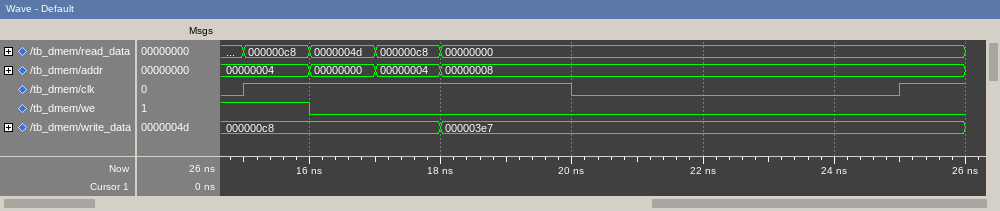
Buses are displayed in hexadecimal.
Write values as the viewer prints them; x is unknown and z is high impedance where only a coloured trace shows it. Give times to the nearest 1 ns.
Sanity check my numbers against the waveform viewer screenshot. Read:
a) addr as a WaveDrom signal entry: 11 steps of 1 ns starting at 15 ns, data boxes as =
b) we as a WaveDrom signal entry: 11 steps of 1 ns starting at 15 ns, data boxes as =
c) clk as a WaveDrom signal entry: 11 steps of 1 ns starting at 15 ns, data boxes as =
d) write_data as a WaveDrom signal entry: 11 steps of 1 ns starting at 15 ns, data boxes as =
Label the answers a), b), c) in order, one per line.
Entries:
a) {name: 'addr', wave: '====.......', data: '00000004 00000000 00000004 00000008'}
b) {name: 'we', wave: '10.........'}
c) {name: 'clk', wave: '1....0....1'}
d) {name: 'write_data', wave: '=..=.......', data: '000000c8 000003e7'}
